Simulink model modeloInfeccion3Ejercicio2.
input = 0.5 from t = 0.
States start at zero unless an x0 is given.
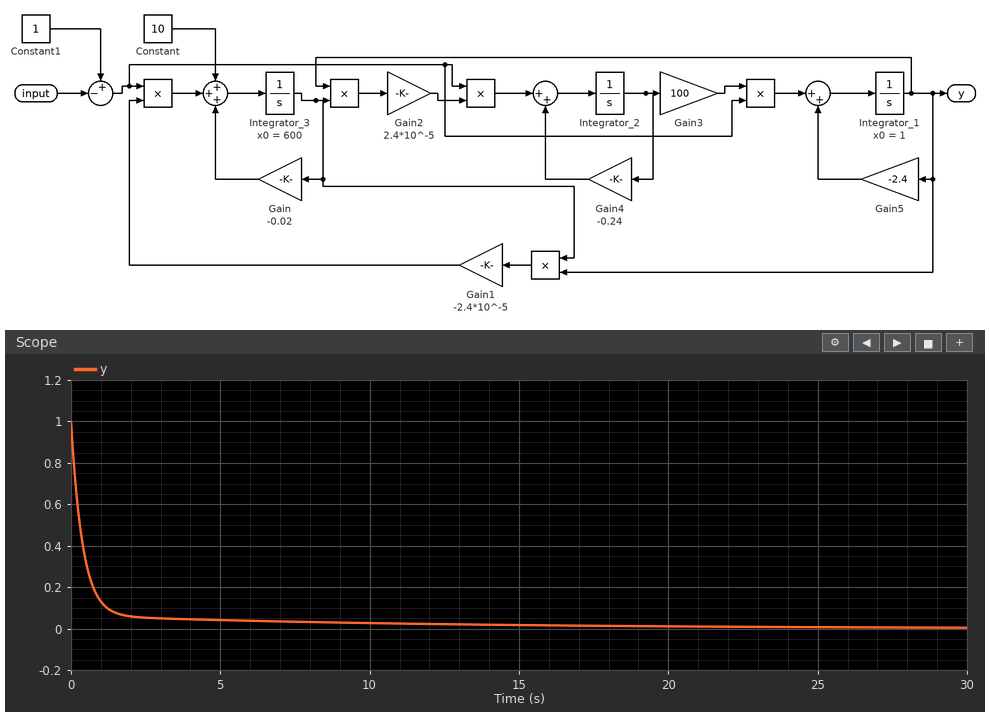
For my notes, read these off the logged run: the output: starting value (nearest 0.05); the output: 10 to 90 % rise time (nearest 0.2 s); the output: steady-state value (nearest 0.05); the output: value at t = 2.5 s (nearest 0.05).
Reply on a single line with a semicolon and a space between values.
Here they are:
1.00; 1.2 s; 0.00; 0.05
